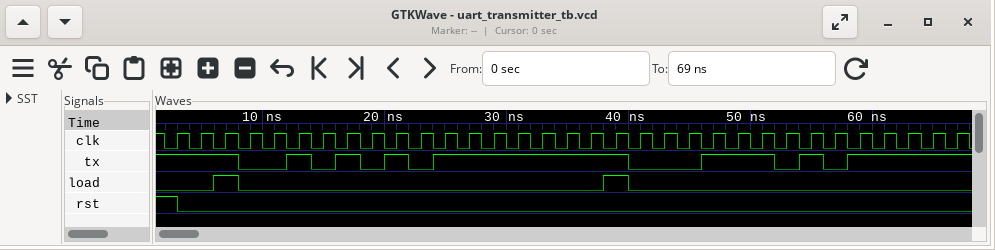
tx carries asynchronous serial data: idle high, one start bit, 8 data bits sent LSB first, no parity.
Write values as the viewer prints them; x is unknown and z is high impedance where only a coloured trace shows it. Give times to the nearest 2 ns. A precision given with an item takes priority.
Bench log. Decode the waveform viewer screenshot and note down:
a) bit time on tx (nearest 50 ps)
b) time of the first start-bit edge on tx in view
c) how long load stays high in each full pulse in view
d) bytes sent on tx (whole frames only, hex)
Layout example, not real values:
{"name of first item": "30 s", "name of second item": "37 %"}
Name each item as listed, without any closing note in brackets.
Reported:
{"bit time on tx": "2000 ps", "time of the first start-bit edge on tx in view": "8 ns", "how long load stays high in each full pulse in view": "2 ns, 2 ns", "bytes sent on tx": "AA, 5C"}
